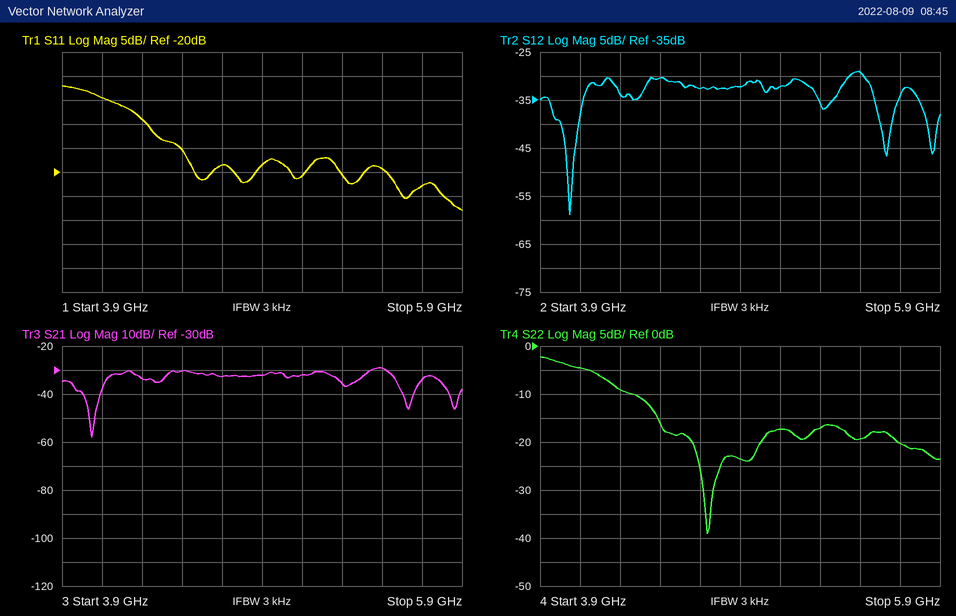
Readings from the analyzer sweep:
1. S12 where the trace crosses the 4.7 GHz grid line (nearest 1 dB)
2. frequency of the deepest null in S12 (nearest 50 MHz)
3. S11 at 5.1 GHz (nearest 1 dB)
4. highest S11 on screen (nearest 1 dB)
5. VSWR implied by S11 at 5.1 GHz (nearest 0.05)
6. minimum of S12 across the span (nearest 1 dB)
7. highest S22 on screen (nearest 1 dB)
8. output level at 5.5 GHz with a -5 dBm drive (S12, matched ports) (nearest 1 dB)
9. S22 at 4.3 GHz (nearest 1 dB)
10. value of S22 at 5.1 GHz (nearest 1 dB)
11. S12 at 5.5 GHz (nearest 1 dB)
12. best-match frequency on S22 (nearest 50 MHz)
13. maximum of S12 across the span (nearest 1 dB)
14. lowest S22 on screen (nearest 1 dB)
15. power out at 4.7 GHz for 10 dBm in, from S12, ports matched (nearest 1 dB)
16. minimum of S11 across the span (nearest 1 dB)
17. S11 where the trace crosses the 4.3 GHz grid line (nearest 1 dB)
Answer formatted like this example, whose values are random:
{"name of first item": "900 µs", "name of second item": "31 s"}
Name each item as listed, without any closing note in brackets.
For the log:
{"S12 where the trace crosses the 4.7 GHz grid line": "-33 dB", "frequency of the deepest null in S12": "4.05 GHz", "S11 at 5.1 GHz": "-21 dB", "highest S11 on screen": "-2 dB", "VSWR implied by S11 at 5.1 GHz": "1.20", "minimum of S12 across the span": "-59 dB", "highest S22 on screen": "-2 dB", "output level at 5.5 GHz with a -5 dBm drive (S12, matched ports)": "-34 dBm", "S22 at 4.3 GHz": "-9 dB", "value of S22 at 5.1 GHz": "-17 dB", "S12 at 5.5 GHz": "-29 dB", "best-match frequency on S22": "4.75 GHz", "maximum of S12 across the span": "-29 dB", "lowest S22 on screen": "-39 dB", "power out at 4.7 GHz for 10 dBm in, from S12, ports matched": "-23 dBm", "minimum of S11 across the span": "-28 dB", "S11 where the trace crosses the 4.3 GHz grid line": "-9 dB"}
